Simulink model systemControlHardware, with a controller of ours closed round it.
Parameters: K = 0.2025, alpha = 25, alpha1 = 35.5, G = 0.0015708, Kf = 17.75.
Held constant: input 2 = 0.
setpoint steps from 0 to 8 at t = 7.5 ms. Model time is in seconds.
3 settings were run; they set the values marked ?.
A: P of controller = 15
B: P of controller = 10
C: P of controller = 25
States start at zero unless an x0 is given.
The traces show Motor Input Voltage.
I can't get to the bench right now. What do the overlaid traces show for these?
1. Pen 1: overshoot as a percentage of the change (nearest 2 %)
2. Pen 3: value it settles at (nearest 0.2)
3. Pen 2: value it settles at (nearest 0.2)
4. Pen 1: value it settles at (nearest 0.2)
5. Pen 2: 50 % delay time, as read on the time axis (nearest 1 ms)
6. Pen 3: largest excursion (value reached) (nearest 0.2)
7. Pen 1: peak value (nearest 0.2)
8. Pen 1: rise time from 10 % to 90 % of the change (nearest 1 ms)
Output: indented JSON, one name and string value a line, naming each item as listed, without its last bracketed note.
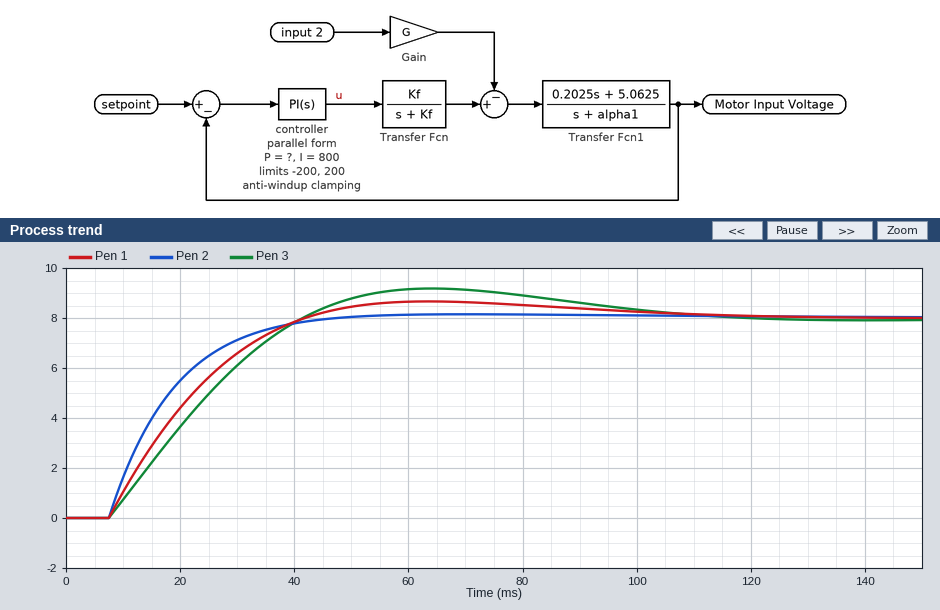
{
  "Pen 1: overshoot as a percentage of the change": "8 %",
  "Pen 3: value it settles at": "8.0",
  "Pen 2: value it settles at": "8.0",
  "Pen 1: value it settles at": "8.0",
  "Pen 2: 50 % delay time, as read on the time axis": "15 ms",
  "Pen 3: largest excursion (value reached)": "9.2",
  "Pen 1: peak value": "8.6",
  "Pen 1: rise time from 10 % to 90 % of the change": "25 ms"
}
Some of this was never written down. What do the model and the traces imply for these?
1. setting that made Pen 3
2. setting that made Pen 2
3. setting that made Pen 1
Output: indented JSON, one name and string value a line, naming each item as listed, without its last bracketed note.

{
  "setting that made Pen 3": "B",
  "setting that made Pen 2": "C",
  "setting that made Pen 1": "A"
}
